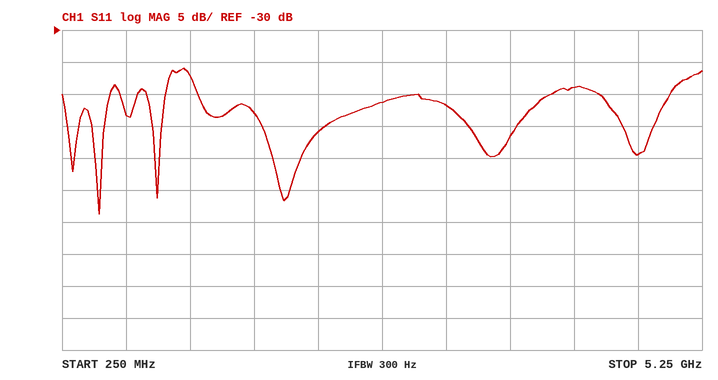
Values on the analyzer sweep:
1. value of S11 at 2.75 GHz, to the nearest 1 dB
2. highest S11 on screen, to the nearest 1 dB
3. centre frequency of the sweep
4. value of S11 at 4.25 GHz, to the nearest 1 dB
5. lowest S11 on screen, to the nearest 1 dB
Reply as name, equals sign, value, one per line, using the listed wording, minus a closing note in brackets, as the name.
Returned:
value of S11 at 2.75 GHz, to the nearest 1 dB = -41 dB
highest S11 on screen, to the nearest 1 dB = -36 dB
centre frequency of the sweep = 2.75 GHz
value of S11 at 4.25 GHz, to the nearest 1 dB = -39 dB
lowest S11 on screen, to the nearest 1 dB = -59 dB
